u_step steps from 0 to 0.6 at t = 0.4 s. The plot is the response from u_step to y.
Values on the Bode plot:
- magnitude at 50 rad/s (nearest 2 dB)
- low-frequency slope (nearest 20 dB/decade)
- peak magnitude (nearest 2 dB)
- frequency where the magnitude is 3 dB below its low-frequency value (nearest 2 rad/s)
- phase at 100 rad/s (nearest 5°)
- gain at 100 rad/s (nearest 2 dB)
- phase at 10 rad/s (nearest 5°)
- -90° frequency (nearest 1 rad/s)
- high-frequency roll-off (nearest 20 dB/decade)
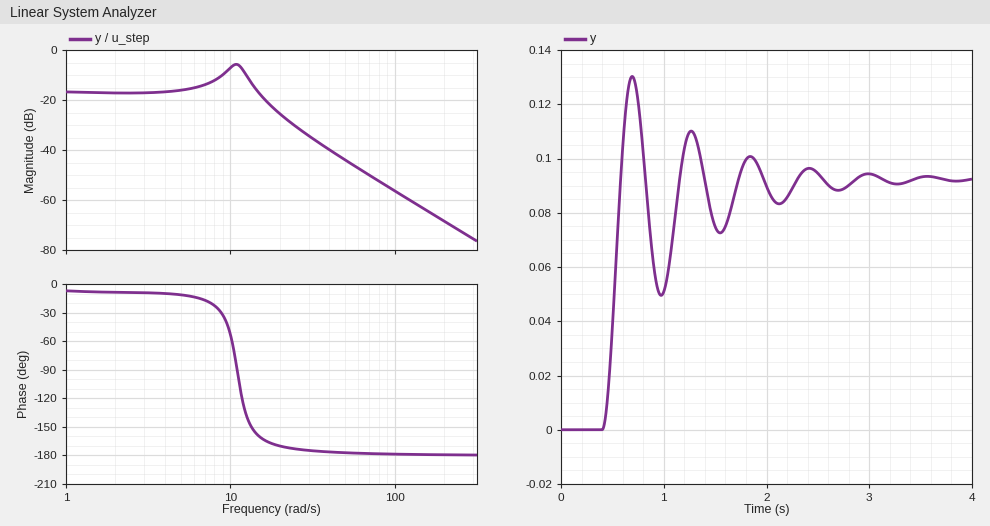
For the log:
-44 dB
0 dB/decade
-6 dB
16 rad/s
-180°
-56 dB
-55°
11 rad/s
-40 dB/decade
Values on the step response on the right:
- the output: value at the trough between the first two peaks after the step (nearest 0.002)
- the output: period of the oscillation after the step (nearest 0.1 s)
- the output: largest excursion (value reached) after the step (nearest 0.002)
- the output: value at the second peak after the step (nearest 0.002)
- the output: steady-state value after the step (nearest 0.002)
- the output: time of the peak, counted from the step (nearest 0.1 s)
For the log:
0.050
0.6 s
0.130
0.110
0.092
0.3 s
